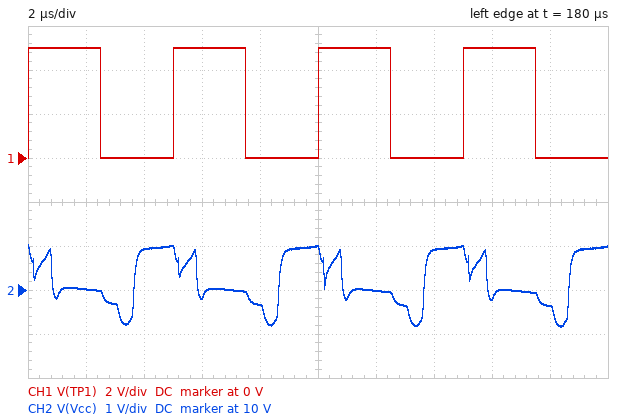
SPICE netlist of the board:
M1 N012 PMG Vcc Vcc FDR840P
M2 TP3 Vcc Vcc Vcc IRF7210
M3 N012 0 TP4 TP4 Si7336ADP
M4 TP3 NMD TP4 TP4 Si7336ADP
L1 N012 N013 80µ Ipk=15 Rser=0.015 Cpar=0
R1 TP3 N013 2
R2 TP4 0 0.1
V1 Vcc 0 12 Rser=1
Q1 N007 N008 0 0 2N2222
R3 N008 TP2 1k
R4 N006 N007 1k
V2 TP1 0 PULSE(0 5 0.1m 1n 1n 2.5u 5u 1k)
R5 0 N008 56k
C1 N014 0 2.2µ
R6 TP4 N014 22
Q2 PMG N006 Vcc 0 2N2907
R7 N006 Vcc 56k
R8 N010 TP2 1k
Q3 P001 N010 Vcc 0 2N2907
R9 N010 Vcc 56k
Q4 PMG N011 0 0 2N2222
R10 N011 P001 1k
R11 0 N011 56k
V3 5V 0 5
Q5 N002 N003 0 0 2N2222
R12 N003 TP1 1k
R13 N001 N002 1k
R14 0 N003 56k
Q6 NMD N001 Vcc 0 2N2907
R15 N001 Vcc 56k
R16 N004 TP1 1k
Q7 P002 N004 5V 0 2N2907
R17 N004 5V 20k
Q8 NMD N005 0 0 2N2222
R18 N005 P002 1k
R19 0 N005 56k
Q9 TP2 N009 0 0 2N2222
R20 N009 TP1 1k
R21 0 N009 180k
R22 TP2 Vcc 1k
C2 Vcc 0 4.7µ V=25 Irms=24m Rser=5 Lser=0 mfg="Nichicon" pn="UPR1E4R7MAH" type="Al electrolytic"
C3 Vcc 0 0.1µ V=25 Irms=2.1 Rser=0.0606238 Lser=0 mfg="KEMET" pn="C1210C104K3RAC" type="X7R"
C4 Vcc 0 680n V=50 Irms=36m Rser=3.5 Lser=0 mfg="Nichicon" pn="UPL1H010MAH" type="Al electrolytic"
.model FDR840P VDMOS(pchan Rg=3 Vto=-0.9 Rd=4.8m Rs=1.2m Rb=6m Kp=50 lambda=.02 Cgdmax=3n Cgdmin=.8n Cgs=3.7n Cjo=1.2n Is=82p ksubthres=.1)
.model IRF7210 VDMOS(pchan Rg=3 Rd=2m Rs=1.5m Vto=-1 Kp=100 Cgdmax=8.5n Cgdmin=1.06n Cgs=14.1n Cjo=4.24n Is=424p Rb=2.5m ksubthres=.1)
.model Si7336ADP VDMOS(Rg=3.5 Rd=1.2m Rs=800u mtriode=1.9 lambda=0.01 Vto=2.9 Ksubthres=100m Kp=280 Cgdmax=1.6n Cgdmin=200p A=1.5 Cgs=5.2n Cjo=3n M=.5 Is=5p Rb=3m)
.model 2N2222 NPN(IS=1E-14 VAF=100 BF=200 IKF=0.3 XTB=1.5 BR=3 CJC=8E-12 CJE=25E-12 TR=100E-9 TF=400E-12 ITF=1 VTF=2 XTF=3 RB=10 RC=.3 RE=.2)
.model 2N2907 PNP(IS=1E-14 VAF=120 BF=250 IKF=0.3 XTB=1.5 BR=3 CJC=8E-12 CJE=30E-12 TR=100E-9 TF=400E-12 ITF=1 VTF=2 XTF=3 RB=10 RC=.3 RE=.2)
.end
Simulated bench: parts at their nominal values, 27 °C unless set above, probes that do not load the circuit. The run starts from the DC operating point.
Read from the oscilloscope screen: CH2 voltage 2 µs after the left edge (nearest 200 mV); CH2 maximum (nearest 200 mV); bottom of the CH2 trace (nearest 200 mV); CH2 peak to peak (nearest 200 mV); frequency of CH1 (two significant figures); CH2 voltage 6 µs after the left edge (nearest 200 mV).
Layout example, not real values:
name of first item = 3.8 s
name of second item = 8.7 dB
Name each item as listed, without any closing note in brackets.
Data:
CH2 voltage 2 µs after the left edge = 10.0 V
CH2 maximum = 11.0 V
bottom of the CH2 trace = 9.2 V
CH2 peak to peak = 1.8 V
frequency of CH1 = 200 kHz
CH2 voltage 6 µs after the left edge = 9.8 V
